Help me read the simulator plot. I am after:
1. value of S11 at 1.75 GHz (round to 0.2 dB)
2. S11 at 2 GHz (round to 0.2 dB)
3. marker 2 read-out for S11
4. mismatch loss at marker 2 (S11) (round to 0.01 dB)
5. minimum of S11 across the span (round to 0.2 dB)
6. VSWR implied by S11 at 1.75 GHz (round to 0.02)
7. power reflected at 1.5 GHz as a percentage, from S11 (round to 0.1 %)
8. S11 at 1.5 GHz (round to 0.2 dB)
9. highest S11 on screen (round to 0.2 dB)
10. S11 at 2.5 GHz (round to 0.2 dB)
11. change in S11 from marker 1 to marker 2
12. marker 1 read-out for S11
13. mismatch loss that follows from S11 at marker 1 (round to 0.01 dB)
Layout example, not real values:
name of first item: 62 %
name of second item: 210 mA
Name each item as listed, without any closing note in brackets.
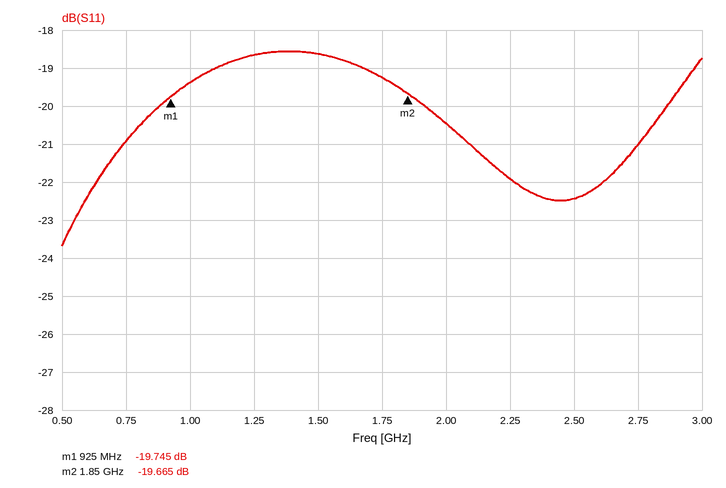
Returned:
value of S11 at 1.75 GHz: -19.2 dB
S11 at 2 GHz: -20.4 dB
marker 2 read-out for S11: -19.665 dB
mismatch loss at marker 2 (S11): 0.05 dB
minimum of S11 across the span: -23.6 dB
VSWR implied by S11 at 1.75 GHz: 1.24
power reflected at 1.5 GHz as a percentage, from S11: 1.4 %
S11 at 1.5 GHz: -18.6 dB
highest S11 on screen: -18.6 dB
S11 at 2.5 GHz: -22.4 dB
change in S11 from marker 1 to marker 2: 0.080 dB
marker 1 read-out for S11: -19.745 dB
mismatch loss that follows from S11 at marker 1: 0.05 dB
